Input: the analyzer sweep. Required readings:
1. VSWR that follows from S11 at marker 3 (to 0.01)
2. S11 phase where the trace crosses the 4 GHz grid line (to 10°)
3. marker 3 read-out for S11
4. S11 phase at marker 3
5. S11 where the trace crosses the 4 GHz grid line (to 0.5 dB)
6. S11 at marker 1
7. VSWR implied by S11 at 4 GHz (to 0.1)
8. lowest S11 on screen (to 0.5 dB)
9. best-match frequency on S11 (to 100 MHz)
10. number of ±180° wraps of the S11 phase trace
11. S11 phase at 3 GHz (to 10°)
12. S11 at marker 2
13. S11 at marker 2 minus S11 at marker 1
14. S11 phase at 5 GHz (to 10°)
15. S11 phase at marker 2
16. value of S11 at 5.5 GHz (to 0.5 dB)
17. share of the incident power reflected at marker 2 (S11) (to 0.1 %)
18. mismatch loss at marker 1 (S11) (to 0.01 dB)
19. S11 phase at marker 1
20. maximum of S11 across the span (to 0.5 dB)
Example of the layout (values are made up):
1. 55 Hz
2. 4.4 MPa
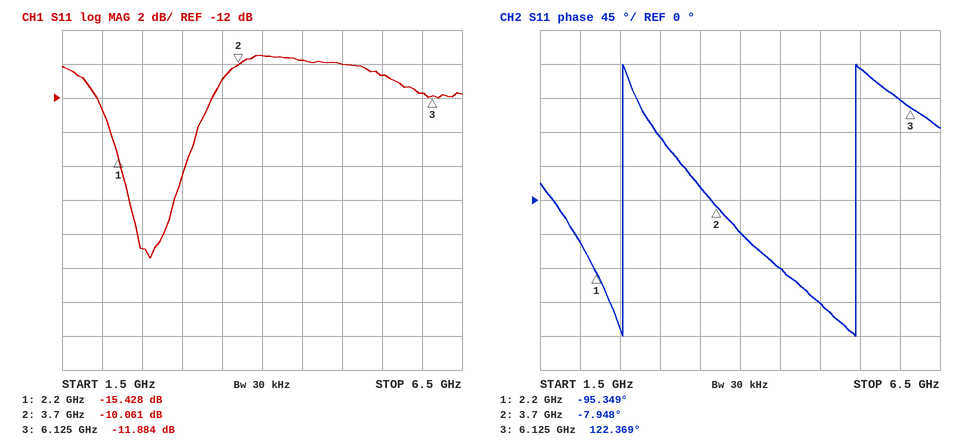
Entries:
1. 1.68
2. -40°
3. -11.884 dB
4. 122.369°
5. -9.5 dB
6. -15.428 dB
7. 2.0
8. -21.5 dB
9. 2.6 GHz
10. 2
11. 80°
12. -10.061 dB
13. 5.367 dB
14. -140°
15. -7.948°
16. -10.5 dB
17. 9.9 %
18. 0.13 dB
19. -95.349°
20. -9.5 dB
